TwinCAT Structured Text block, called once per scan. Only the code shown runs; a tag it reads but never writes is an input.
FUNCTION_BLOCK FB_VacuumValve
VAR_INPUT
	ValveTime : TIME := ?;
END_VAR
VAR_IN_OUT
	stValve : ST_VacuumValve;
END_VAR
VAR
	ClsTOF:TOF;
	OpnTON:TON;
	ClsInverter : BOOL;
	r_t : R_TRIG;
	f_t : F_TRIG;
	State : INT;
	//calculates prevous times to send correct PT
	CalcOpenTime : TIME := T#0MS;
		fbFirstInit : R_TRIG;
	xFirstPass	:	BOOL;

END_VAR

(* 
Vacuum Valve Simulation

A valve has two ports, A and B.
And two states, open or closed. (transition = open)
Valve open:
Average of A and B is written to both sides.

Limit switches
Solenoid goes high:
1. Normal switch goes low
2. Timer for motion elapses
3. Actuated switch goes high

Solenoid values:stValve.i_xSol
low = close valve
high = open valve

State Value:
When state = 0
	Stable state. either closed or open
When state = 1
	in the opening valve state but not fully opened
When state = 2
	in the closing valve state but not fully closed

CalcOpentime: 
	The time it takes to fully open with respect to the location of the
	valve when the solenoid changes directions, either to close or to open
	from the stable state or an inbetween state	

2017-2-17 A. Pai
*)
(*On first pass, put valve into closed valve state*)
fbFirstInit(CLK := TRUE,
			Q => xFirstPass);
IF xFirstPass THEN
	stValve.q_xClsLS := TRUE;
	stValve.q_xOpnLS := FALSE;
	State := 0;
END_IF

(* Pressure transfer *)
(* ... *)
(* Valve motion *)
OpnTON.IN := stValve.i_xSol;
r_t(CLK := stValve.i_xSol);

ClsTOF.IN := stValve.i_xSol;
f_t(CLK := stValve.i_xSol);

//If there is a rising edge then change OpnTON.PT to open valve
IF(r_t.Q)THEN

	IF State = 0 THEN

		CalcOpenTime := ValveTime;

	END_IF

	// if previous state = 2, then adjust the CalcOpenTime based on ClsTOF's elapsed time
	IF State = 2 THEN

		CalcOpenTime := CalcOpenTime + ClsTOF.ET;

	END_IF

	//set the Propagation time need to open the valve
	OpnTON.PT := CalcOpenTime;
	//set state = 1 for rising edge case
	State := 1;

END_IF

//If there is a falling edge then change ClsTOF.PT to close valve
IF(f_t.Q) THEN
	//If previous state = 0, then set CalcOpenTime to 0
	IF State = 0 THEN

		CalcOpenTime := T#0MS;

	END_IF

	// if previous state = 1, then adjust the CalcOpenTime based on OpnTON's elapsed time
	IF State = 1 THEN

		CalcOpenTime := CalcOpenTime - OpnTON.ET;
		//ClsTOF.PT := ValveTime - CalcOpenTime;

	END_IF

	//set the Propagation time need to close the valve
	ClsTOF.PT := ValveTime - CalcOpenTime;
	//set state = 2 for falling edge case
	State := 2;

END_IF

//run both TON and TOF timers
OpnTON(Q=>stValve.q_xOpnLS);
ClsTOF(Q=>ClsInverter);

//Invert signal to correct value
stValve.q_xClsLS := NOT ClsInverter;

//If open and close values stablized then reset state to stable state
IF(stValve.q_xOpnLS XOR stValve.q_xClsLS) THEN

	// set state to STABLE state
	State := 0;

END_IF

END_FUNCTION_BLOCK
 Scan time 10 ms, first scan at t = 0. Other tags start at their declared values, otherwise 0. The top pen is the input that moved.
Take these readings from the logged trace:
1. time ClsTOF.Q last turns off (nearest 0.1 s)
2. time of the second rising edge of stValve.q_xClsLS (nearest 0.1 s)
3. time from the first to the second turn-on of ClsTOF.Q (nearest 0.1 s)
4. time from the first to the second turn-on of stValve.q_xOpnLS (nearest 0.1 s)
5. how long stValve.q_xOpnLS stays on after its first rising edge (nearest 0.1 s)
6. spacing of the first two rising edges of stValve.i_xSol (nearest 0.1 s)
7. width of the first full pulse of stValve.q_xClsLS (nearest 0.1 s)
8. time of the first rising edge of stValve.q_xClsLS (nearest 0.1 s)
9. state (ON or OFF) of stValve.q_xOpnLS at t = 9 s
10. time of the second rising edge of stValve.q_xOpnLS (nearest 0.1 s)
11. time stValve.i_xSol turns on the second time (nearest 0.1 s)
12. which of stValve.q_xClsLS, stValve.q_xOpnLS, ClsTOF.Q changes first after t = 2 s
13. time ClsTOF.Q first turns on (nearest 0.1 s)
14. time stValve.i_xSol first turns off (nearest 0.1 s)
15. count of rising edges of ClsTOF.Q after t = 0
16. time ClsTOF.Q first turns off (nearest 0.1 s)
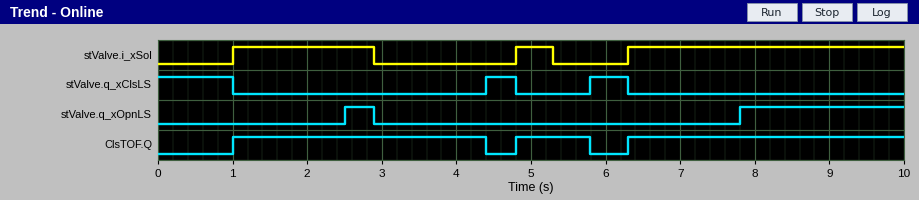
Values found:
5.8 s
5.8 s
3.8 s
5.3 s
0.4 s
3.8 s
0.4 s
4.4 s
ON
7.8 s
4.8 s
stValve.q_xOpnLS
1.0 s
2.9 s
3
4.4 s
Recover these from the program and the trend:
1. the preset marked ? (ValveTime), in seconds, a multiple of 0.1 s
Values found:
1.5 s
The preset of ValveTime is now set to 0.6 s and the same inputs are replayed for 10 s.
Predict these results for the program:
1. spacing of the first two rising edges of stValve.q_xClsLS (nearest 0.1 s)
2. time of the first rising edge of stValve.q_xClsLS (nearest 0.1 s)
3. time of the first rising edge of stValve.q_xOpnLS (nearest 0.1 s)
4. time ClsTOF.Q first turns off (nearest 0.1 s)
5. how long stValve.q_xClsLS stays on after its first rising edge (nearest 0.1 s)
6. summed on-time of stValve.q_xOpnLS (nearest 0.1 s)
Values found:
2.3 s
3.5 s
1.6 s
3.5 s
1.3 s
4.4 s
